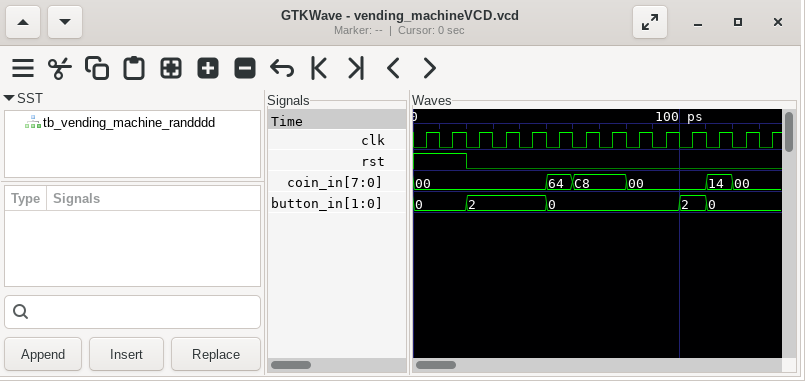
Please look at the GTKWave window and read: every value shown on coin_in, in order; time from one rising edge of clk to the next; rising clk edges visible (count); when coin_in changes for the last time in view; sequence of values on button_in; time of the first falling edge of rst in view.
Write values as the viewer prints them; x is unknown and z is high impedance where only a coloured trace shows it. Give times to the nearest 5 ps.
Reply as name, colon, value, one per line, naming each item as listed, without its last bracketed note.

every value shown on coin_in, in order: 00, 64, C8, 00, 14, 00
time from one rising edge of clk to the next: 10 ps
rising clk edges visible: 14
when coin_in changes for the last time in view: 120 ps
sequence of values on button_in: 0, 2, 0, 2, 0
time of the first falling edge of rst in view: 20 ps
